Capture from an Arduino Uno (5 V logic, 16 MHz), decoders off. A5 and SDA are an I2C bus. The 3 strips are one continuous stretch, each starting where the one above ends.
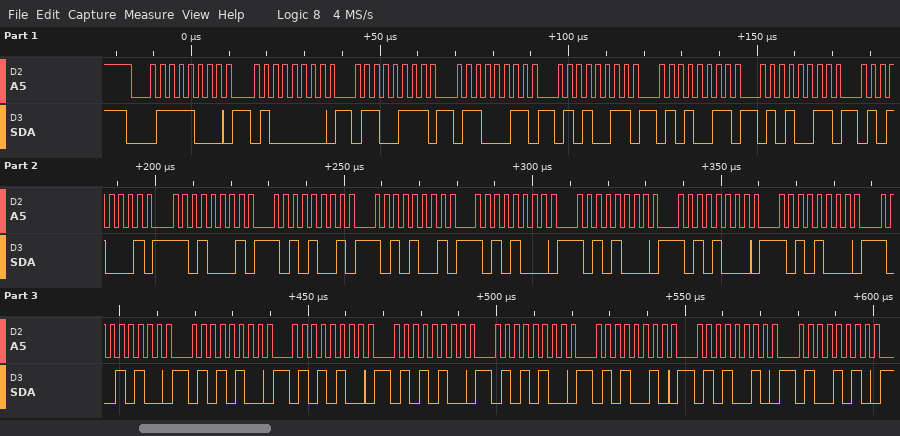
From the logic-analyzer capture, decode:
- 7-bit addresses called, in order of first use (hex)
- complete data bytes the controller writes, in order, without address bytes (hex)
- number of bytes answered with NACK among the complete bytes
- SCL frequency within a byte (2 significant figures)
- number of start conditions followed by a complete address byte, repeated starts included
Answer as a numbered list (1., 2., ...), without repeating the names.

1. 0x3C
2. 40 67 63 53 53 53 51 D1 A9 A9 A8 A8 A8 A8 94 54 54 54 54 52 52 4A
3. 0
4. 400 kHz
5. 1
